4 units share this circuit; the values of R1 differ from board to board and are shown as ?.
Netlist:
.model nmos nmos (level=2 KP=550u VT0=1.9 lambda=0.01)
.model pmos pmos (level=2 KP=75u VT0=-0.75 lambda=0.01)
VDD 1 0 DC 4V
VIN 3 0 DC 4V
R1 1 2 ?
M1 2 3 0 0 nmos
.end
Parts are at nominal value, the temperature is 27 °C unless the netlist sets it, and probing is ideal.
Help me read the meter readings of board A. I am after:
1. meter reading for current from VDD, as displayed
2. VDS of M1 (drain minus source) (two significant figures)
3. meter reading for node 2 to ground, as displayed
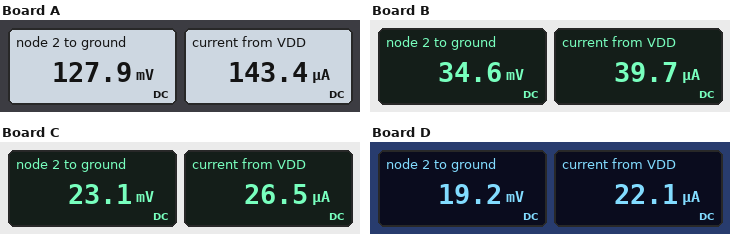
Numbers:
143.4 µA
130 mV
127.9 mV
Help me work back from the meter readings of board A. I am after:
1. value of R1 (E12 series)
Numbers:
27 kΩ
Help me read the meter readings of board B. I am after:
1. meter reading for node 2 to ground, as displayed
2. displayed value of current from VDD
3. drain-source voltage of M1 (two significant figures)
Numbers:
34.6 mV
39.7 µA
35 mV
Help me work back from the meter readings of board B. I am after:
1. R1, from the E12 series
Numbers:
100 kΩ
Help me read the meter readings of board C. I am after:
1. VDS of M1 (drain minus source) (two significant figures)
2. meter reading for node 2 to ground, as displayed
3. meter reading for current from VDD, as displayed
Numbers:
23 mV
23.1 mV
26.5 µA
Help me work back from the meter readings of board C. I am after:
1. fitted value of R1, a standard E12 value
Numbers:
150 kΩ
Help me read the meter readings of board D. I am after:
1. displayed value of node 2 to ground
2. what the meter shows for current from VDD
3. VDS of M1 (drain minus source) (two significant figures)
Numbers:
19.2 mV
22.1 µA
19 mV
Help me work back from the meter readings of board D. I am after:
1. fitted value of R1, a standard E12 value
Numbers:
180 kΩ
